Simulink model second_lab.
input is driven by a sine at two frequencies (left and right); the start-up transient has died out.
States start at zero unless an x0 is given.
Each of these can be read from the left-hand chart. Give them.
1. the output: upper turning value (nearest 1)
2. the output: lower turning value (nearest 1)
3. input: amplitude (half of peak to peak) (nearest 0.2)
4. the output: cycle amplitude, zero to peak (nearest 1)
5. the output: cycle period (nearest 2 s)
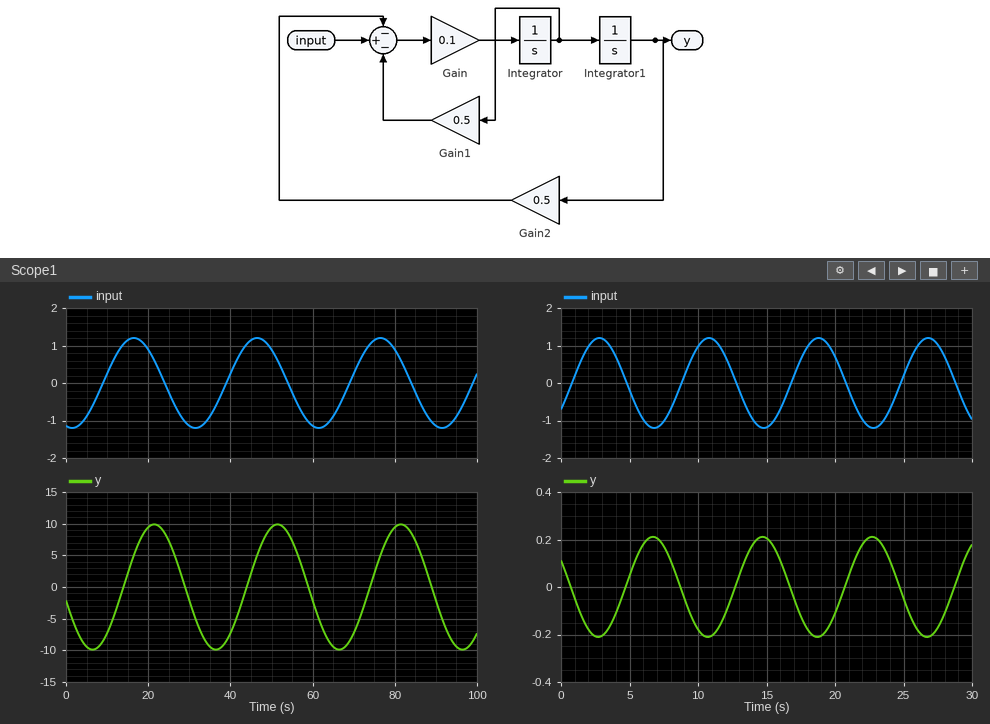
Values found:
10
-10
1.2
10
30 s
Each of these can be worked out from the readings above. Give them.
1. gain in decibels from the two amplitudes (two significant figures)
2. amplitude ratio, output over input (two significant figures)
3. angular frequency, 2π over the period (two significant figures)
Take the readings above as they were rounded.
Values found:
18 dB
8.3
0.21 rad/s
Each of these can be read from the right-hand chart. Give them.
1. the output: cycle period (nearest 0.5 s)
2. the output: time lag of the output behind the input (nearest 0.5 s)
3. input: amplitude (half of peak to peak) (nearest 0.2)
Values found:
8.0 s
4.0 s
1.2
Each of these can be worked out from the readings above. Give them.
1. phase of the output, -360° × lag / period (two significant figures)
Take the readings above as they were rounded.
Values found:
-180°
